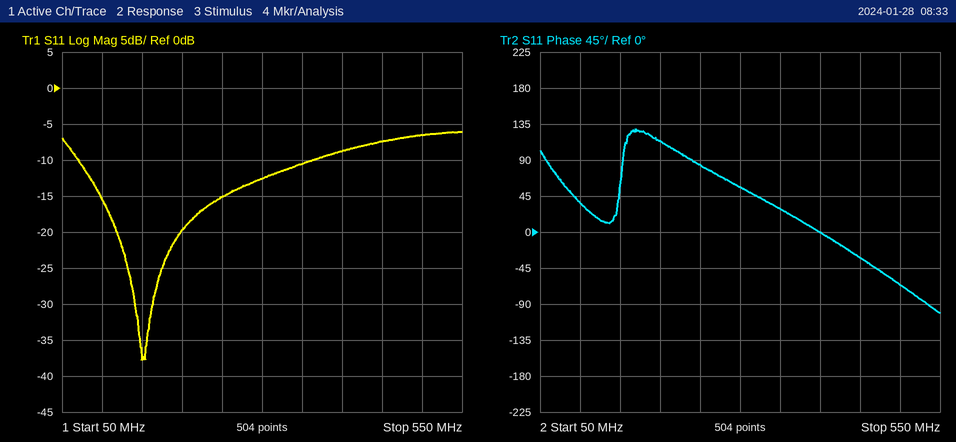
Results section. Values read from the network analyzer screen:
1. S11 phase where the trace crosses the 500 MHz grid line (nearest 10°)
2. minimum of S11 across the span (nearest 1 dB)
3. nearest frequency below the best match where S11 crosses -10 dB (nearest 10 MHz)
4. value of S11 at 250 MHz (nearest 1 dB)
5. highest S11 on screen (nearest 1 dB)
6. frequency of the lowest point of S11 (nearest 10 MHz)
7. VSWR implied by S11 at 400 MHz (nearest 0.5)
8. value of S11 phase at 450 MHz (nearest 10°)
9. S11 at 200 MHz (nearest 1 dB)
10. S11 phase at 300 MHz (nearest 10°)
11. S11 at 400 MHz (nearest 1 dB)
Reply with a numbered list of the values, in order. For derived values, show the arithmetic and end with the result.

1. -70°
2. -38 dB
3. 70 MHz
4. -15 dB
5. -6 dB
6. 150 MHz
7. |Γ| = 10^(-9/20) = 0.3548; VSWR = (1 + 0.3548)/(1 − 0.3548) ≈ 2.10, so 2.0 to the nearest 0.5
8. -30°
9. -20 dB
10. 60°
11. -9 dB
